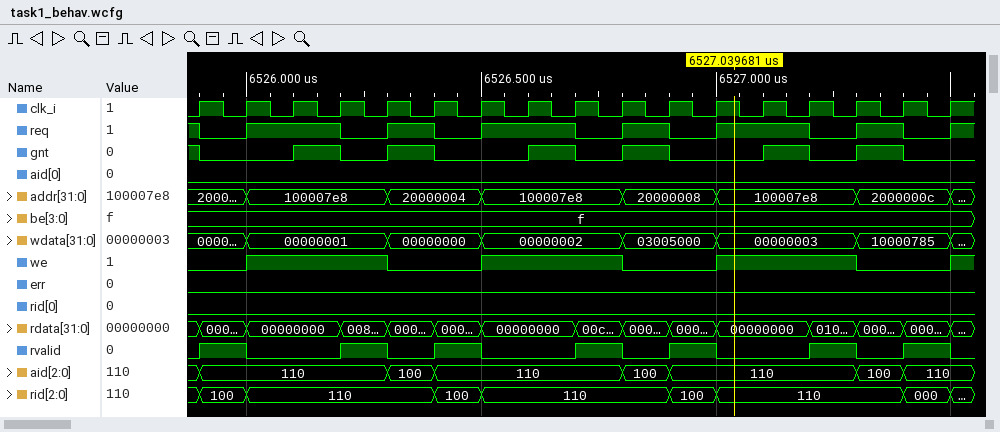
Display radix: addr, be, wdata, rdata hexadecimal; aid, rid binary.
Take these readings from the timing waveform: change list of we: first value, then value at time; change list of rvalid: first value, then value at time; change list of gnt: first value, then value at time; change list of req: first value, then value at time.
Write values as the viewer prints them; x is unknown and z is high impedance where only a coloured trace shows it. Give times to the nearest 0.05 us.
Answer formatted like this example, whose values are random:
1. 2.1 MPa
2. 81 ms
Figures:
1. 0, 1 at 6526 us, 0 at 6526.3 us, 1 at 6526.5 us, 0 at 6526.8 us, 1 at 6527 us, 0 at 6527.3 us, 1 at 6527.5 us
2. 0, 1 at 6525.9 us, 0 at 6526 us, 1 at 6526.2 us, 0 at 6526.3 us, 1 at 6526.4 us, 0 at 6526.5 us, 1 at 6526.7 us, 0 at 6526.8 us, 1 at 6526.9 us, 0 at 6527 us, 1 at 6527.2 us, 0 at 6527.3 us, 1 at 6527.4 us, 0 at 6527.5 us
3. 1, 0 at 6525.9 us, 1 at 6526.1 us, 0 at 6526.2 us, 1 at 6526.3 us, 0 at 6526.4 us, 1 at 6526.6 us, 0 at 6526.7 us, 1 at 6526.8 us, 0 at 6526.9 us, 1 at 6527.1 us, 0 at 6527.2 us, 1 at 6527.3 us, 0 at 6527.4 us
4. 1, 0 at 6525.9 us, 1 at 6526 us, 0 at 6526.2 us, 1 at 6526.3 us, 0 at 6526.4 us, 1 at 6526.5 us, 0 at 6526.7 us, 1 at 6526.8 us, 0 at 6526.9 us, 1 at 6527 us, 0 at 6527.2 us, 1 at 6527.3 us, 0 at 6527.4 us, 1 at 6527.5 us
